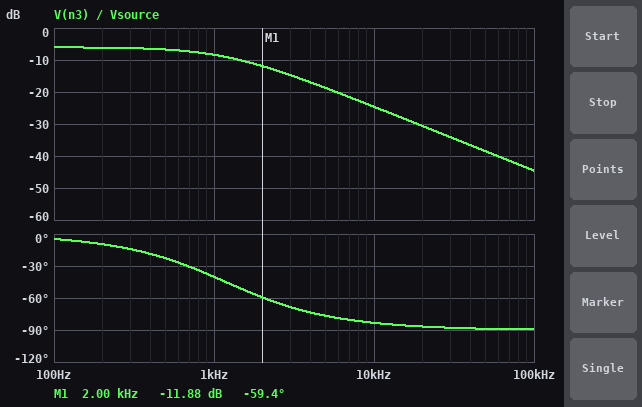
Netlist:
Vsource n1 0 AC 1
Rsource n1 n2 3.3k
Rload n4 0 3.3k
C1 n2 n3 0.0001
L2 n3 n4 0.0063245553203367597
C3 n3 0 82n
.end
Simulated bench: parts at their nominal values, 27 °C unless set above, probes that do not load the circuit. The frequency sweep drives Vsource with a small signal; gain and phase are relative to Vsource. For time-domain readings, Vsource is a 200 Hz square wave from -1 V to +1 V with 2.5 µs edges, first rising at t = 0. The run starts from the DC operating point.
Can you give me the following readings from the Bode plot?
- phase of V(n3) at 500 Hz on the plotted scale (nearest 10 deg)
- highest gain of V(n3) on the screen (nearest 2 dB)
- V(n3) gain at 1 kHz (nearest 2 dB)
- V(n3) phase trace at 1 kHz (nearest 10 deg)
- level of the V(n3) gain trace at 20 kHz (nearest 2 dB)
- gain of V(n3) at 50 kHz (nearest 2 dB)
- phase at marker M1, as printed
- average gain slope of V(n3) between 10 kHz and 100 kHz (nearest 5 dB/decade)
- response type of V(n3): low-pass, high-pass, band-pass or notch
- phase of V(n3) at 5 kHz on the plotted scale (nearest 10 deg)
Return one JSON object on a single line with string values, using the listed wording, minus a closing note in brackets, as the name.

{"phase of V(n3) at 500 Hz on the plotted scale": "-20 deg", "highest gain of V(n3) on the screen": "-6 dB", "V(n3) gain at 1 kHz": "-8 dB", "V(n3) phase trace at 1 kHz": "-40 deg", "level of the V(n3) gain trace at 20 kHz": "-30 dB", "gain of V(n3) at 50 kHz": "-38 dB", "phase at marker M1, as printed": "-59.4 deg", "average gain slope of V(n3) between 10 kHz and 100 kHz": "-20 dB/decade", "response type of V(n3): low-pass, high-pass, band-pass or notch": "low-pass", "phase of V(n3) at 5 kHz on the plotted scale": "-80 deg"}
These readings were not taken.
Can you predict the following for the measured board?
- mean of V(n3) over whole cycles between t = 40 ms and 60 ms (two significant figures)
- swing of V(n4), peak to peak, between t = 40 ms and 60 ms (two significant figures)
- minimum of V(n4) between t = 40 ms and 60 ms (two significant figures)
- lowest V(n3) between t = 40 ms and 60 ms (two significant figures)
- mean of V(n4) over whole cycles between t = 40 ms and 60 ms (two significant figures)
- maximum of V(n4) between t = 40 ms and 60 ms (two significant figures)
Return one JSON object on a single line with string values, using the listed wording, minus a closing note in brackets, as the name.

{"mean of V(n3) over whole cycles between t = 40 ms and 60 ms": "460 mV", "swing of V(n4), peak to peak, between t = 40 ms and 60 ms": "1.0 V", "minimum of V(n4) between t = 40 ms and 60 ms": "-43 mV", "lowest V(n3) between t = 40 ms and 60 ms": "-43 mV", "mean of V(n4) over whole cycles between t = 40 ms and 60 ms": "460 mV", "maximum of V(n4) between t = 40 ms and 60 ms": "970 mV"}
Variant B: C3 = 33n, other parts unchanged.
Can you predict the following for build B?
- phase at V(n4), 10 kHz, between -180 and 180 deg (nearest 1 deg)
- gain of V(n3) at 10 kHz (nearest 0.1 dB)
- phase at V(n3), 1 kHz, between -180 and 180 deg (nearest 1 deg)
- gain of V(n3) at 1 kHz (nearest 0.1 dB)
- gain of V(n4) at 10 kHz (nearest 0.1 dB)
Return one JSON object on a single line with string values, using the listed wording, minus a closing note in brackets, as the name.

{"phase at V(n4), 10 kHz, between -180 and 180 deg": "-80 deg", "gain of V(n3) at 10 kHz": "-16.9 dB", "phase at V(n3), 1 kHz, between -180 and 180 deg": "-19 deg", "gain of V(n3) at 1 kHz": "-6.5 dB", "gain of V(n4) at 10 kHz": "-17.0 dB"}
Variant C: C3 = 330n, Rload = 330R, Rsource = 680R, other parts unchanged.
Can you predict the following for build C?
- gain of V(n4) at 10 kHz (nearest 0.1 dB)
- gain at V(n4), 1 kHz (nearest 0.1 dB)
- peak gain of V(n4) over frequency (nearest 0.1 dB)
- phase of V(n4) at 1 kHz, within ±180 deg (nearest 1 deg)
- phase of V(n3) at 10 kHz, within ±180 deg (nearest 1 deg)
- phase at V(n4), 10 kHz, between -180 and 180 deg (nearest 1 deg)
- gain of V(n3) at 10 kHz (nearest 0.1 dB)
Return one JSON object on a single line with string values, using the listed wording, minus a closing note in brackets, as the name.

{"gain of V(n4) at 10 kHz": "-26.3 dB", "gain at V(n4), 1 kHz": "-10.3 dB", "peak gain of V(n4) over frequency": "-9.7 dB", "phase of V(n4) at 1 kHz, within ±180 deg": "-28 deg", "phase of V(n3) at 10 kHz, within ±180 deg": "-82 deg", "phase at V(n4), 10 kHz, between -180 and 180 deg": "-132 deg", "gain of V(n3) at 10 kHz": "-22.4 dB"}
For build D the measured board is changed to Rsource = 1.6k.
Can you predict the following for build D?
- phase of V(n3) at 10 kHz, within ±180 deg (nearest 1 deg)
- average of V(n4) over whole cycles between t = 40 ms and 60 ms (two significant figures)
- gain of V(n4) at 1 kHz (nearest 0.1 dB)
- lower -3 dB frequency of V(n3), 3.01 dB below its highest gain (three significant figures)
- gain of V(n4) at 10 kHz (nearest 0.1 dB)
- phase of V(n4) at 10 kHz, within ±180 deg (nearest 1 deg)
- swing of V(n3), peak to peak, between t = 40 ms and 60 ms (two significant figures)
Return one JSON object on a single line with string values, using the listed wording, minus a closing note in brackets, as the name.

{"phase of V(n3) at 10 kHz, within ±180 deg": "-80 deg", "average of V(n4) over whole cycles between t = 40 ms and 60 ms": "610 mV", "gain of V(n4) at 1 kHz": "-4.6 dB", "lower -3 dB frequency of V(n3), 3.01 dB below its highest gain": "325 mHz", "gain of V(n4) at 10 kHz": "-18.5 dB", "phase of V(n4) at 10 kHz, within ±180 deg": "-87 deg", "swing of V(n3), peak to peak, between t = 40 ms and 60 ms": "1.4 V"}
